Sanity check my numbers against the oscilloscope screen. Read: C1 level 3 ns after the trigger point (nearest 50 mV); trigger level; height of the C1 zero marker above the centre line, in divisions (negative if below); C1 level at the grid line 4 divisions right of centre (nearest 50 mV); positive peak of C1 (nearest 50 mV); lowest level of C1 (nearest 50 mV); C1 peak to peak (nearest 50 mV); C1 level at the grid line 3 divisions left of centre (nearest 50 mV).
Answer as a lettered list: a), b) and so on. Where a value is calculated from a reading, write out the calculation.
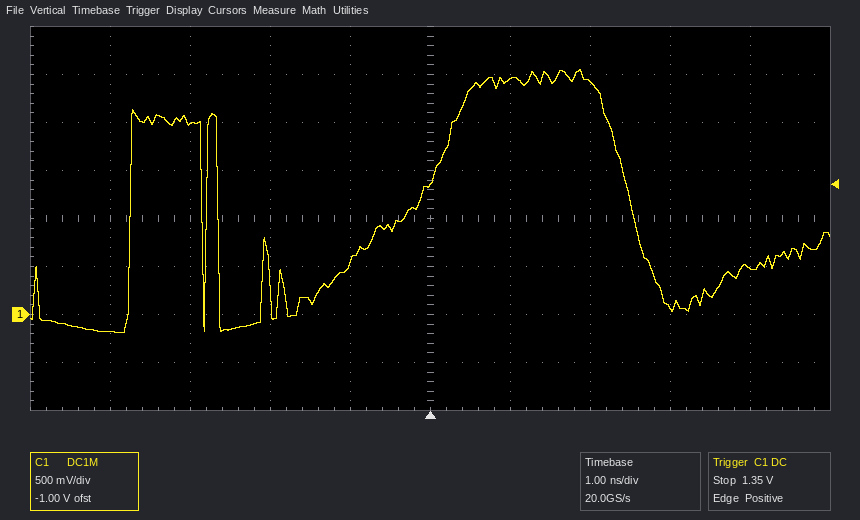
a) 50 mV
b) 1.35 V
c) -2.0 div
d) 500 mV
e) 2.55 V
f) -200 mV
g) 2.55 V − (-200 mV) = 2.75 V
h) 2.00 V
